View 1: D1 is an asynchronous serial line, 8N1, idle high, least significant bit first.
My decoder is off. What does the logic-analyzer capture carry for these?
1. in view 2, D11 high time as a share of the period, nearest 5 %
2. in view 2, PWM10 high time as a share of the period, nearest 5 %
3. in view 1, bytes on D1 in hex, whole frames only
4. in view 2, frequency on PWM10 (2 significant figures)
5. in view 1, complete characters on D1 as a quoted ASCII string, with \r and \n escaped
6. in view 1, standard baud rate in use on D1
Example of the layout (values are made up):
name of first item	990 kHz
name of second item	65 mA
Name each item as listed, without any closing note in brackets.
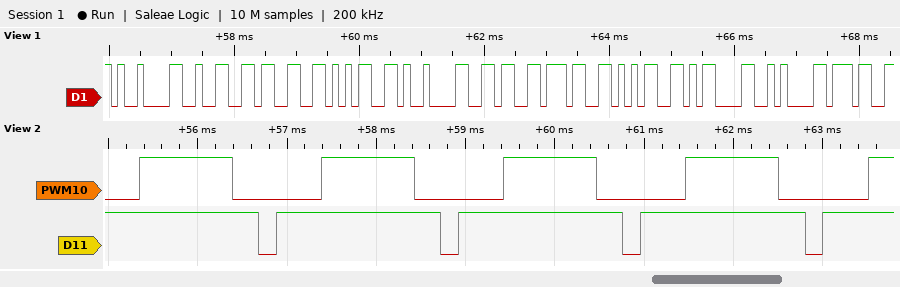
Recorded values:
in view 2, D11 high time as a share of the period, nearest 5 %	90 %
in view 2, PWM10 high time as a share of the period, nearest 5 %	50 %
in view 1, bytes on D1 in hex, whole frames only	09 32 33 35 09 36 37 35 0D 0A 37
in view 2, frequency on PWM10	490 Hz
in view 1, complete characters on D1 as a quoted ASCII string, with \r and \n escaped	"\t235\t675\r\n7"
in view 1, standard baud rate in use on D1	9600 baud
